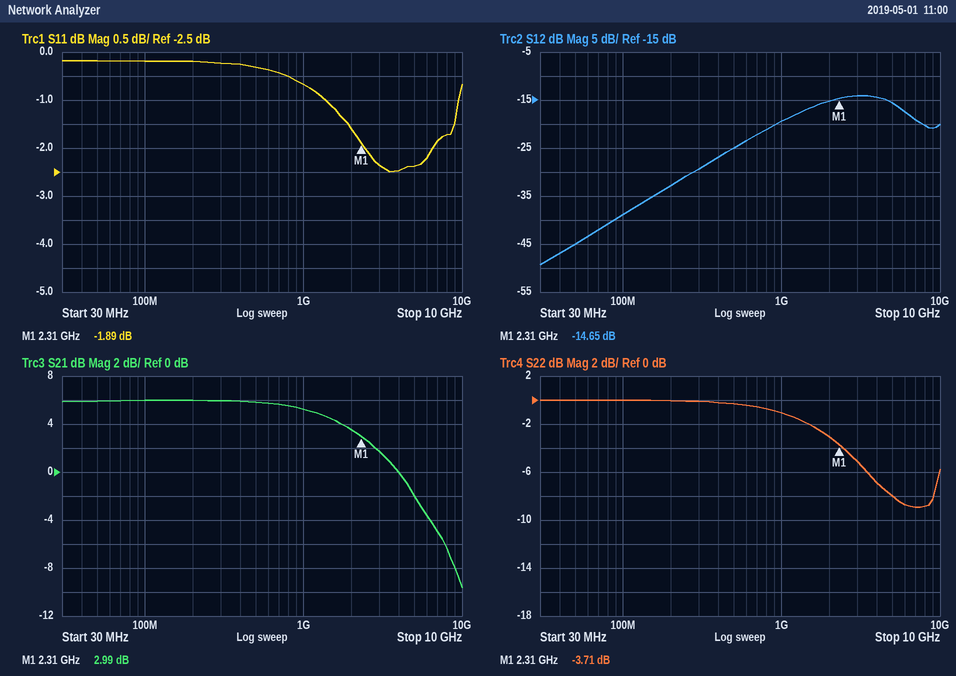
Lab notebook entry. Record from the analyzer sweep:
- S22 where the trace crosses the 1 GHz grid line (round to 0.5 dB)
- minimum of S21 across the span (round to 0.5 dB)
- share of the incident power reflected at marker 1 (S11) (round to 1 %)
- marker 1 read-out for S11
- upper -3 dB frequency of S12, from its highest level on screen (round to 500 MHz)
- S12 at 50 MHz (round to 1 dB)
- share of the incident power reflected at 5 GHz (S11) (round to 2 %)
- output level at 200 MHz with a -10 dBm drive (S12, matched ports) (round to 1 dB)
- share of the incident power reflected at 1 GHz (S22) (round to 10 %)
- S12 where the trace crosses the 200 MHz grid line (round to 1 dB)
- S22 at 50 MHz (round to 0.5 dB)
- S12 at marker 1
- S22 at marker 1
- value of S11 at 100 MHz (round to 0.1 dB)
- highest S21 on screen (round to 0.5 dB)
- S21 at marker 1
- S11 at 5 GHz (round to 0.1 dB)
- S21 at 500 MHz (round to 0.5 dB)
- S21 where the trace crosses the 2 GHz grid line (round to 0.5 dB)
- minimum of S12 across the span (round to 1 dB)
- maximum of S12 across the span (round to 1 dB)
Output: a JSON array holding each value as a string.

["-1.0 dB", "-9.5 dB", "65 %", "-1.89 dB", "6.0 GHz", "-45 dB", "58 %", "-43 dBm", "80 %", "-33 dB", "0.0 dB", "-14.65 dB", "-3.71 dB", "-0.2 dB", "6.0 dB", "2.99 dB", "-2.4 dB", "6.0 dB", "3.5 dB", "-49 dB", "-14 dB"]
